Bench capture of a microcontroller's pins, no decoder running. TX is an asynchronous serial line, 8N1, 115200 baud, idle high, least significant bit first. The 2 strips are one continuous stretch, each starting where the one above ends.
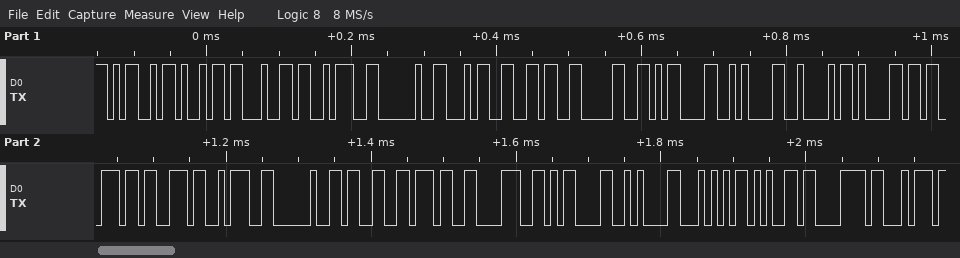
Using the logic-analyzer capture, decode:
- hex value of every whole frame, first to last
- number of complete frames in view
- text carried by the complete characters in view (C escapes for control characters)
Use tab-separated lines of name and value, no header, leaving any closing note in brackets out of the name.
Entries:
hex value of every whole frame, first to last	0x4D 0x69 0x64 0x3A 0x20 0x34 0x36 0x30 0x0D 0x0A 0x42 0x61 0x73 0x73 0x3A 0x20 0x33 0x37 0x38 0x0D 0x0A 0x54 0x65 0x78 0x74
number of complete frames in view	25
text carried by the complete characters in view	"Mid: 460\r\nBass: 378\r\nText"
